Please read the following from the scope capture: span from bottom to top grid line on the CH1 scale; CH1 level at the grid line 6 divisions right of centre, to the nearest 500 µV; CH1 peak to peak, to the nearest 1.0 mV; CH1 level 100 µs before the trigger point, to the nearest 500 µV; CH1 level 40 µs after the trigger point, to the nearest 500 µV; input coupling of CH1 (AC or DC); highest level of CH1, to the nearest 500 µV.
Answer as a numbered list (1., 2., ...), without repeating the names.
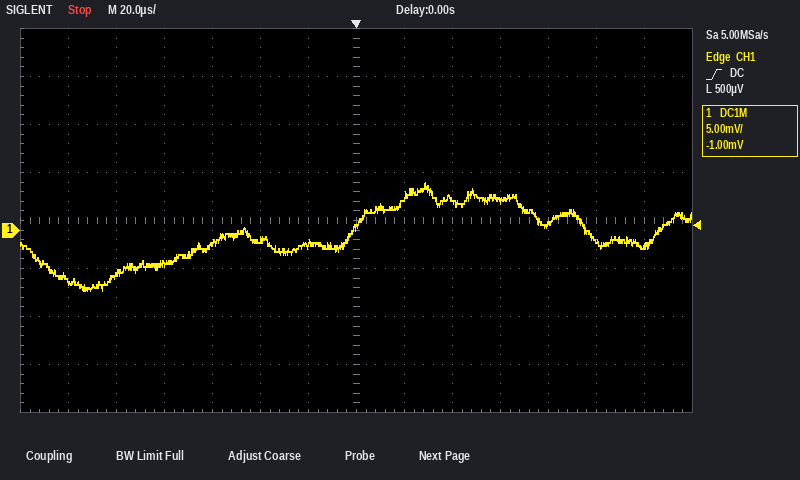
1. 40 mV
2. -1.5 mV
3. 11.0 mV
4. -4.5 mV
5. 3.0 mV
6. DC
7. 5.0 mV
